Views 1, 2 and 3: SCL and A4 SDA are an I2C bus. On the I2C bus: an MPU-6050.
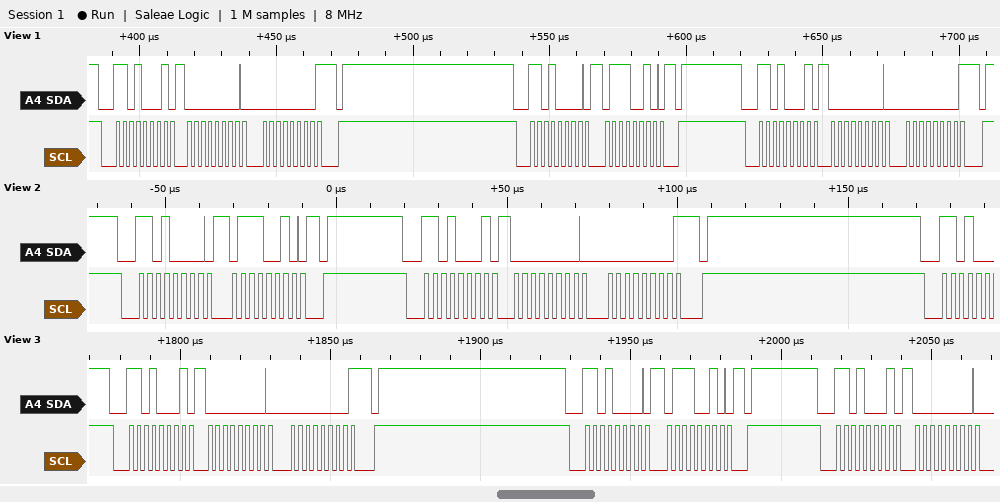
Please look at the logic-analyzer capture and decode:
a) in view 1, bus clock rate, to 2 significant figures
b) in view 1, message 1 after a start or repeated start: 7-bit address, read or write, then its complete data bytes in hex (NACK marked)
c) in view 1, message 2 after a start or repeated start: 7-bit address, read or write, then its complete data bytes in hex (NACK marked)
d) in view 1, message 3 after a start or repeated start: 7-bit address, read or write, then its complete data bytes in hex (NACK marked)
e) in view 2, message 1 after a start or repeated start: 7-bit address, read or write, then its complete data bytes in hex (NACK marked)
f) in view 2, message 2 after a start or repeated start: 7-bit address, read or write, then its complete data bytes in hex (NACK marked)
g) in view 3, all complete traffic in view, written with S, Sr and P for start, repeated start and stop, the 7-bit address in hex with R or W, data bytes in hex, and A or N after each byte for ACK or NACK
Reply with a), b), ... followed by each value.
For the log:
a) 400 kHz
b) 0x68 read: 00 00 NACK
c) 0x68 write: 72
d) 0x68 read: 00 00 NACK
e) 0x68 write: 72
f) 0x68 read: 00 00 NACK
g) S 68R A 00 A 00 N P S 68W A 72 A P S 68R A 00 A
